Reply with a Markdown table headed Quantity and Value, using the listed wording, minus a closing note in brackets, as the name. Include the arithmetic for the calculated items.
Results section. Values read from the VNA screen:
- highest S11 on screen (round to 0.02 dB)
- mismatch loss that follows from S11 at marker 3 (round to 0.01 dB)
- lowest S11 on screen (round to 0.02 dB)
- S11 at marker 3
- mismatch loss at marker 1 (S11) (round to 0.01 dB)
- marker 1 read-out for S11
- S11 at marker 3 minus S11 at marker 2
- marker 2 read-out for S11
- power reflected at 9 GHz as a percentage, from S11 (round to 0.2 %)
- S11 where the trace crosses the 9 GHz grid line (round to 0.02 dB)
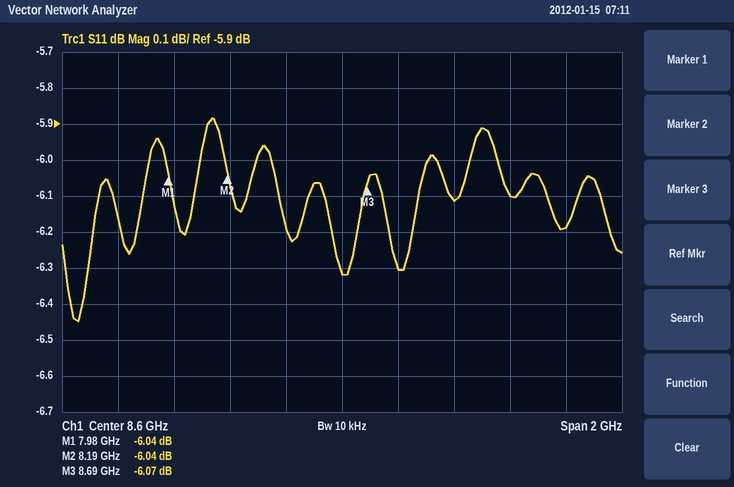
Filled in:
| Quantity | Value |
|---|---|
| highest S11 on screen | -5.88 dB |
| mismatch loss that follows from S11 at marker 3 | −10 log10(1 − 10^(-6.07/10)) ≈ 1.23 dB |
| lowest S11 on screen | -6.44 dB |
| S11 at marker 3 | -6.07 dB |
| mismatch loss at marker 1 (S11) | −10 log10(1 − 10^(-6.04/10)) ≈ 1.24 dB |
| marker 1 read-out for S11 | -6.04 dB |
| S11 at marker 3 minus S11 at marker 2 | -6.07 − (-6.04) = -0.03 dB |
| marker 2 read-out for S11 | -6.04 dB |
| power reflected at 9 GHz as a percentage, from S11 | 10^(-6.12/10) ≈ 24.4 % |
| S11 where the trace crosses the 9 GHz grid line | -6.12 dB |
